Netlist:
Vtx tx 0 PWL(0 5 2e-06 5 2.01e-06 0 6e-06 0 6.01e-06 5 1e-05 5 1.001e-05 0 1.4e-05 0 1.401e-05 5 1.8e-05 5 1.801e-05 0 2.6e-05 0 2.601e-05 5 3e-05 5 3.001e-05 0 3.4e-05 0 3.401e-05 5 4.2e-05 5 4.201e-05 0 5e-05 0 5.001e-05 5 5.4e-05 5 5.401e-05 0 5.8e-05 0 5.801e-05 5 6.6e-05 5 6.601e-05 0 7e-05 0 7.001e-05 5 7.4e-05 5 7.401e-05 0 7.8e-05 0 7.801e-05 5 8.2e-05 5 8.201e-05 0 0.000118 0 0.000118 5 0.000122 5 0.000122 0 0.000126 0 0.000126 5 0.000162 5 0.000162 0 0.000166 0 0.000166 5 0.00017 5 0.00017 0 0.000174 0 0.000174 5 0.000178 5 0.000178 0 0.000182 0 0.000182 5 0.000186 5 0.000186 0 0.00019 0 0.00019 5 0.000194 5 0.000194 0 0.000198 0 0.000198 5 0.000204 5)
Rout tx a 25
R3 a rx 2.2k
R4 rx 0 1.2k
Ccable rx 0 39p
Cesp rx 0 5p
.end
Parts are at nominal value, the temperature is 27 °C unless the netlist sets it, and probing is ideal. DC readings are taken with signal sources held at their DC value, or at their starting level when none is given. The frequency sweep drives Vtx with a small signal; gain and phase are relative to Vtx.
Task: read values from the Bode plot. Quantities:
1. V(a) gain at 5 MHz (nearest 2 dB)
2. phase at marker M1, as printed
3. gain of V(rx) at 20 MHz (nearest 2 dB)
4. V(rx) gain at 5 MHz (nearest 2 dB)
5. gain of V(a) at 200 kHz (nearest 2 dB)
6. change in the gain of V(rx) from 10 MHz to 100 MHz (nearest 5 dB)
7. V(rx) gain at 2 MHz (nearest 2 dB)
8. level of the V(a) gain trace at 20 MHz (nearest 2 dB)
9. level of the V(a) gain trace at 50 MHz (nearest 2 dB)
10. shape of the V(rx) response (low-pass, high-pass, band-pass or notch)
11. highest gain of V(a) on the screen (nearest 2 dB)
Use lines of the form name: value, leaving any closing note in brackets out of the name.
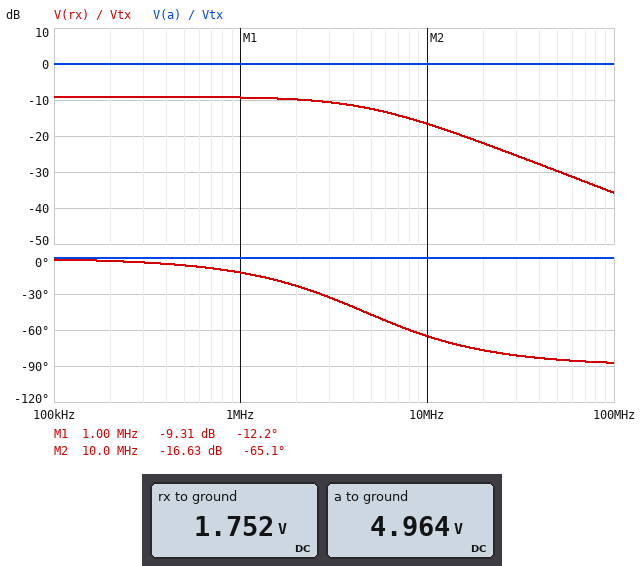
V(a) gain at 5 MHz: 0 dB
phase at marker M1, as printed: -12.2 deg
gain of V(rx) at 20 MHz: -22 dB
V(rx) gain at 5 MHz: -12 dB
gain of V(a) at 200 kHz: 0 dB
change in the gain of V(rx) from 10 MHz to 100 MHz: -20 dB
V(rx) gain at 2 MHz: -10 dB
level of the V(a) gain trace at 20 MHz: 0 dB
level of the V(a) gain trace at 50 MHz: 0 dB
shape of the V(rx) response: low-pass
highest gain of V(a) on the screen: 0 dB
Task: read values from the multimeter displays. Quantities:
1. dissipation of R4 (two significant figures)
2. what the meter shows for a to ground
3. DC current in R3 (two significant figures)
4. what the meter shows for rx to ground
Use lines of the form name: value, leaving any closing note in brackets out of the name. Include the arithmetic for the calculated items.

dissipation of R4: (1.752 V)^2 / 1.2 kΩ = 2.6 mW
what the meter shows for a to ground: 4.964 V
DC current in R3: (4.964 V - 1.752 V) / 2.2 kΩ = 1.5 mA
what the meter shows for rx to ground: 1.752 V
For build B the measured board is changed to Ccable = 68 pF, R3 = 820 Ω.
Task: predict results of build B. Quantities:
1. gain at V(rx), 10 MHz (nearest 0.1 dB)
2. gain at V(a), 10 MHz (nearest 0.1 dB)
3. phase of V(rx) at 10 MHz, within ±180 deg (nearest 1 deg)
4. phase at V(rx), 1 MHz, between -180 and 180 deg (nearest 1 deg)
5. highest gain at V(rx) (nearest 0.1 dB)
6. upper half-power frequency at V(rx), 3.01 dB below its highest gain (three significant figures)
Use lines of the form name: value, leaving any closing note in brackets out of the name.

gain at V(rx), 10 MHz: -12.5 dB
gain at V(a), 10 MHz: -0.2 dB
phase of V(rx) at 10 MHz, within ±180 deg: -66 deg
phase at V(rx), 1 MHz, between -180 and 180 deg: -13 deg
highest gain at V(rx): -4.6 dB
upper half-power frequency at V(rx), 3.01 dB below its highest gain: 4.40 MHz
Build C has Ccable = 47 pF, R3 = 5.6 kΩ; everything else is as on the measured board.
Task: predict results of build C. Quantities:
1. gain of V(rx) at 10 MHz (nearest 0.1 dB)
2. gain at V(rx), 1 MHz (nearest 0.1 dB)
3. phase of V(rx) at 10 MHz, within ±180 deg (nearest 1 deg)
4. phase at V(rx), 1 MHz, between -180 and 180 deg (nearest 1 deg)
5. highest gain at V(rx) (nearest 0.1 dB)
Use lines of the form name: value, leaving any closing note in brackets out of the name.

gain of V(rx) at 10 MHz: -25.7 dB
gain at V(rx), 1 MHz: -15.5 dB
phase of V(rx) at 10 MHz, within ±180 deg: -73 deg
phase at V(rx), 1 MHz, between -180 and 180 deg: -18 deg
highest gain at V(rx): -15.1 dB
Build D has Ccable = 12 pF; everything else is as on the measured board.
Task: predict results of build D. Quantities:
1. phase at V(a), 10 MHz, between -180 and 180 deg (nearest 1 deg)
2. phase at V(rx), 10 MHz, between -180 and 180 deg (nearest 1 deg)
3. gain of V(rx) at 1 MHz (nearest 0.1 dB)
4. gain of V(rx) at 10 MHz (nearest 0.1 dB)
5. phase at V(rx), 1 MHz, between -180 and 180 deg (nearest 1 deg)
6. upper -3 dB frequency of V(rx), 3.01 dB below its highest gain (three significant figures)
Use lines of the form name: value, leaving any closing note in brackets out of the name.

phase at V(a), 10 MHz, between -180 and 180 deg: 0 deg
phase at V(rx), 10 MHz, between -180 and 180 deg: -40 deg
gain of V(rx) at 1 MHz: -9.1 dB
gain of V(rx) at 10 MHz: -11.4 dB
phase at V(rx), 1 MHz, between -180 and 180 deg: -5 deg
upper -3 dB frequency of V(rx), 3.01 dB below its highest gain: 12.0 MHz
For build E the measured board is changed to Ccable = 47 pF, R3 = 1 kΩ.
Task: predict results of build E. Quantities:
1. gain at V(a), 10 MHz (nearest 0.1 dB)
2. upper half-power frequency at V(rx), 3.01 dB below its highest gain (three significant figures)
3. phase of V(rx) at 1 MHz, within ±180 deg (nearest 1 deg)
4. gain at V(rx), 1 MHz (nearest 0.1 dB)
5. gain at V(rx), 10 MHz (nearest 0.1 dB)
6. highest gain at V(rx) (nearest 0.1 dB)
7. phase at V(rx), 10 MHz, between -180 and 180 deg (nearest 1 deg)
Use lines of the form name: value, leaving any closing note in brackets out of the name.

gain at V(a), 10 MHz: -0.2 dB
upper half-power frequency at V(rx), 3.01 dB below its highest gain: 5.54 MHz
phase of V(rx) at 1 MHz, within ±180 deg: -10 deg
gain at V(rx), 1 MHz: -5.5 dB
gain at V(rx), 10 MHz: -11.7 dB
highest gain at V(rx): -5.4 dB
phase at V(rx), 10 MHz, between -180 and 180 deg: -61 deg
